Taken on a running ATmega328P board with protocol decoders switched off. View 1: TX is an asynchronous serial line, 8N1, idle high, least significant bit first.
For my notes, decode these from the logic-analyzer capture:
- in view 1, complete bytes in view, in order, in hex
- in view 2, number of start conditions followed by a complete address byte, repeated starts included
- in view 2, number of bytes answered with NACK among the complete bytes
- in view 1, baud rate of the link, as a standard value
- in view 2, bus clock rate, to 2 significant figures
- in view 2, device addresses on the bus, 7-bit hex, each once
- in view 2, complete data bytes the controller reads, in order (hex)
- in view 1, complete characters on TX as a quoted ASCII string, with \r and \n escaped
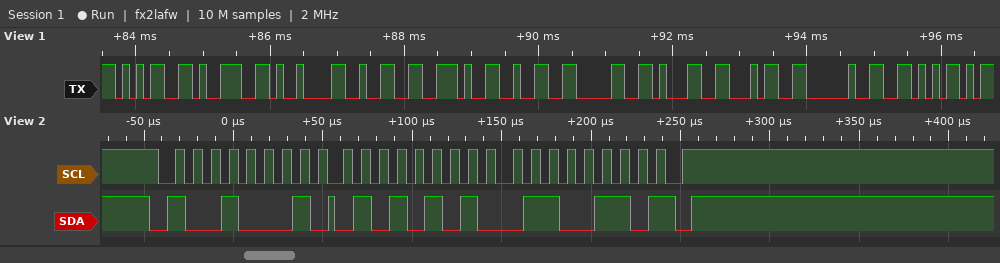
35 39 09 32 2E 32 30 31 34 20 56
1
1
9600 baud
100 kHz
0x48
55 66
"59\t2.2014 V"
